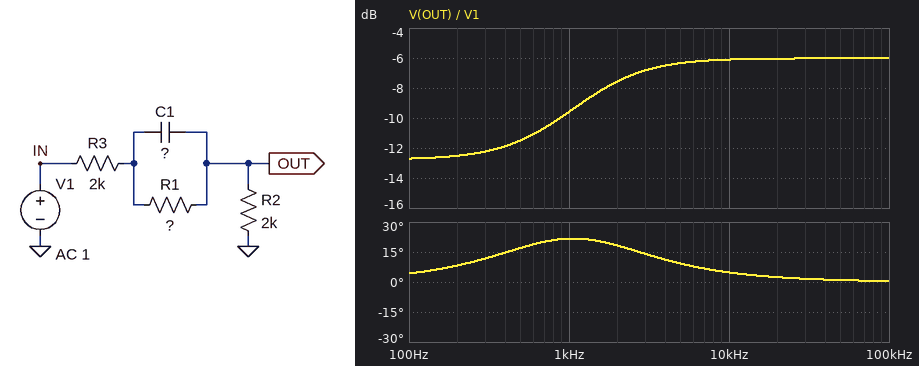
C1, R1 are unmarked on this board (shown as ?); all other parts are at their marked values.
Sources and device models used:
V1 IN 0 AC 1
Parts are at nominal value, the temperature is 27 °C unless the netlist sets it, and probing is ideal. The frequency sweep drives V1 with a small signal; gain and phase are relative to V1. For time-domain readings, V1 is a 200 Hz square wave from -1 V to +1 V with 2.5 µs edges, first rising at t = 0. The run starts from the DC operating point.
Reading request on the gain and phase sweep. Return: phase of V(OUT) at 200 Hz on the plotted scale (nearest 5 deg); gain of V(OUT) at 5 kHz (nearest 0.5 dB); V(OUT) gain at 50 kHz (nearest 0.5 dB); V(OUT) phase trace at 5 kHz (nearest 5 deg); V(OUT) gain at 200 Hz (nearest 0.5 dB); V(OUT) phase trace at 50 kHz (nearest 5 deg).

10 deg
-6.5 dB
-6.0 dB
10 deg
-12.5 dB
0 deg
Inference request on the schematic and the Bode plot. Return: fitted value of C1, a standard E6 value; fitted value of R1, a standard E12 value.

47 nF
4.7 kΩ
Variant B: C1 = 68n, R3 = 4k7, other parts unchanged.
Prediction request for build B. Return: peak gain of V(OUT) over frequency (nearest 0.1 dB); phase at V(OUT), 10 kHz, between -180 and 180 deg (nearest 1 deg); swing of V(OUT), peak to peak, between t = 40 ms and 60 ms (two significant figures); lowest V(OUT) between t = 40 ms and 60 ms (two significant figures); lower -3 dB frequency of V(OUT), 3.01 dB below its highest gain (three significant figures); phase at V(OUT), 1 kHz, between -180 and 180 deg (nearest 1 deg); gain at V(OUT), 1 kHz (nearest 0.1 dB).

-10.5 dB
2 deg
840 mV
-420 mV
471 Hz
14 deg
-11.9 dB
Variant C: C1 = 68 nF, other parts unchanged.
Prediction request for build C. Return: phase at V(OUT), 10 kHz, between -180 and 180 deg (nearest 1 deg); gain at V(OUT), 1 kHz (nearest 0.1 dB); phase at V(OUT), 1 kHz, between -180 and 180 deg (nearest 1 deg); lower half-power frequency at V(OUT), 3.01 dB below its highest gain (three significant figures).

3 deg
-8.4 dB
21 deg
823 Hz
